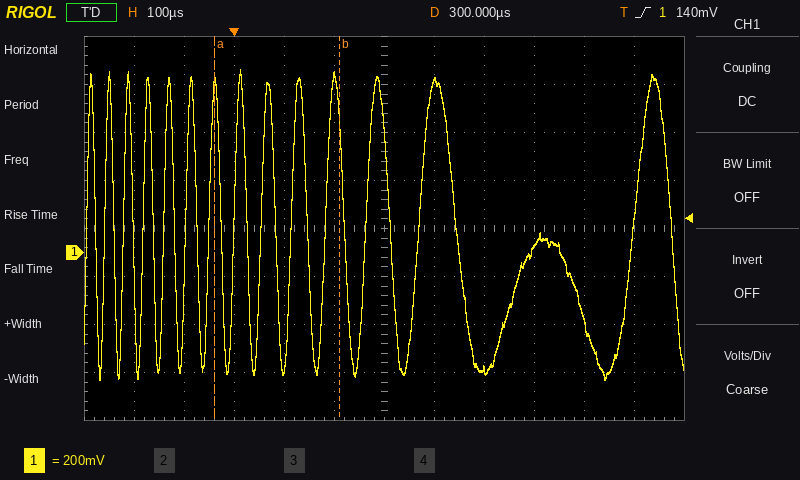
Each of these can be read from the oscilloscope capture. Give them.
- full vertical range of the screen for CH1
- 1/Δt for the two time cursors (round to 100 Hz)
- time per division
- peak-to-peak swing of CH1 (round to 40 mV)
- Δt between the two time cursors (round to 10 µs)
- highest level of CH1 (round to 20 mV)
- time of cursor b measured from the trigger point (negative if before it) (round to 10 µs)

1.6 V
4.0 kHz
100 µs
1.28 V
250 µs
760 mV
+210 µs
